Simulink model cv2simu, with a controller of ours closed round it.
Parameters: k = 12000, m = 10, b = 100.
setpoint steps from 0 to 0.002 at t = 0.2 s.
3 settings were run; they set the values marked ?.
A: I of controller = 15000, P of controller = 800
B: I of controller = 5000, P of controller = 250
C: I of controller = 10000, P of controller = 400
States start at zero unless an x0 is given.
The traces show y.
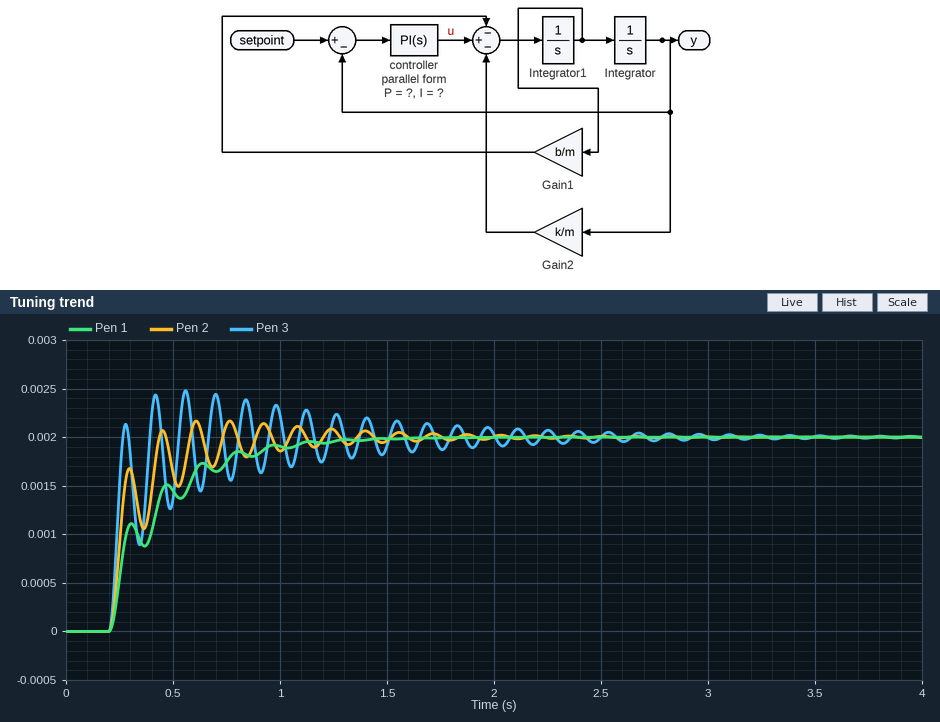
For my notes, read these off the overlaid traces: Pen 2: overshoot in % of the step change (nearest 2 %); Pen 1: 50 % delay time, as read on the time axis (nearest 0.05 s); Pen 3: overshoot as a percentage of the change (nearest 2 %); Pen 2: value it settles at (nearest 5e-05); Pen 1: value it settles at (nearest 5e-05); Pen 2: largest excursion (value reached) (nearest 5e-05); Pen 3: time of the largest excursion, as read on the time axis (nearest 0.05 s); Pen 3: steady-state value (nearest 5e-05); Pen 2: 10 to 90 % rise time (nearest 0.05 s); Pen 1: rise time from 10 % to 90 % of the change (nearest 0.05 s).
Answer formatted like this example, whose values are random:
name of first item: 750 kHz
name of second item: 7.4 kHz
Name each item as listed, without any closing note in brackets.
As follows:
Pen 2: overshoot in % of the step change: 8 %
Pen 1: 50 % delay time, as read on the time axis: 0.30 s
Pen 3: overshoot as a percentage of the change: 24 %
Pen 2: value it settles at: 0.00200
Pen 1: value it settles at: 0.00200
Pen 2: largest excursion (value reached): 0.00215
Pen 3: time of the largest excursion, as read on the time axis: 0.55 s
Pen 3: steady-state value: 0.00200
Pen 2: 10 to 90 % rise time: 0.20 s
Pen 1: rise time from 10 % to 90 % of the change: 0.55 s
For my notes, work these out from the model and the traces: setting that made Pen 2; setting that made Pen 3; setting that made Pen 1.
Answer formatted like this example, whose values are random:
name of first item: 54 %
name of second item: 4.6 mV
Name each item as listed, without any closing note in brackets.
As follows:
setting that made Pen 2: C
setting that made Pen 3: A
setting that made Pen 1: B
